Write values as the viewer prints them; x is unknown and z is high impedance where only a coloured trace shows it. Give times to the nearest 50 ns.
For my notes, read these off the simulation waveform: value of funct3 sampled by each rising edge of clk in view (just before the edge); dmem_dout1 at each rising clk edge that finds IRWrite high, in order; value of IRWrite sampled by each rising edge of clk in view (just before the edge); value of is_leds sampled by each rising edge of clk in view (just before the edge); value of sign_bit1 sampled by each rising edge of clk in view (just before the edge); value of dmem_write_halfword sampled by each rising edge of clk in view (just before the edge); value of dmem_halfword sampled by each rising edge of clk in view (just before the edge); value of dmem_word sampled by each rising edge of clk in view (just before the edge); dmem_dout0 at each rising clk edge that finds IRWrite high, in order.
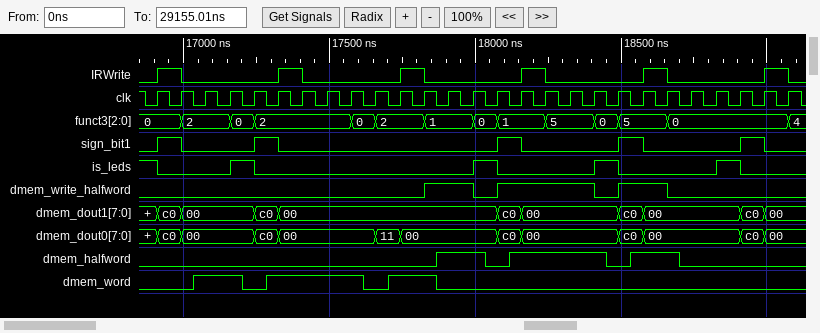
0, 0, 2, 2, 0, 2, 2, 2, 2, 0, 2, 2, 1, 1, 0, 1, 1, 5, 5, 0, 5, 5, 0, 0, 0, 0, 0
c0, 00, 00, 00, 00, 00
0 1 0 0 0 0 1 0 0 0 0 1 0 0 0 0 1 0 0 0 0 1 0 0 0 0 1
1 0 0 0 1 0 0 0 0 0 0 0 0 0 1 0 0 0 0 1 0 0 0 0 1 0 0
0 1 0 0 0 1 0 0 0 0 0 0 0 0 0 1 0 0 0 0 1 0 0 0 0 1 0
0 0 0 0 0 0 0 0 0 0 0 0 1 1 0 1 1 1 1 0 1 1 0 0 0 0 0
0 0 0 0 0 0 0 0 0 0 0 0 1 1 0 1 1 1 1 0 1 1 0 0 0 0 0
0 0 1 1 0 1 1 1 1 0 1 1 0 0 0 0 0 0 0 0 0 0 0 0 0 0 0
c0, 00, 00, 00, 00, 00
